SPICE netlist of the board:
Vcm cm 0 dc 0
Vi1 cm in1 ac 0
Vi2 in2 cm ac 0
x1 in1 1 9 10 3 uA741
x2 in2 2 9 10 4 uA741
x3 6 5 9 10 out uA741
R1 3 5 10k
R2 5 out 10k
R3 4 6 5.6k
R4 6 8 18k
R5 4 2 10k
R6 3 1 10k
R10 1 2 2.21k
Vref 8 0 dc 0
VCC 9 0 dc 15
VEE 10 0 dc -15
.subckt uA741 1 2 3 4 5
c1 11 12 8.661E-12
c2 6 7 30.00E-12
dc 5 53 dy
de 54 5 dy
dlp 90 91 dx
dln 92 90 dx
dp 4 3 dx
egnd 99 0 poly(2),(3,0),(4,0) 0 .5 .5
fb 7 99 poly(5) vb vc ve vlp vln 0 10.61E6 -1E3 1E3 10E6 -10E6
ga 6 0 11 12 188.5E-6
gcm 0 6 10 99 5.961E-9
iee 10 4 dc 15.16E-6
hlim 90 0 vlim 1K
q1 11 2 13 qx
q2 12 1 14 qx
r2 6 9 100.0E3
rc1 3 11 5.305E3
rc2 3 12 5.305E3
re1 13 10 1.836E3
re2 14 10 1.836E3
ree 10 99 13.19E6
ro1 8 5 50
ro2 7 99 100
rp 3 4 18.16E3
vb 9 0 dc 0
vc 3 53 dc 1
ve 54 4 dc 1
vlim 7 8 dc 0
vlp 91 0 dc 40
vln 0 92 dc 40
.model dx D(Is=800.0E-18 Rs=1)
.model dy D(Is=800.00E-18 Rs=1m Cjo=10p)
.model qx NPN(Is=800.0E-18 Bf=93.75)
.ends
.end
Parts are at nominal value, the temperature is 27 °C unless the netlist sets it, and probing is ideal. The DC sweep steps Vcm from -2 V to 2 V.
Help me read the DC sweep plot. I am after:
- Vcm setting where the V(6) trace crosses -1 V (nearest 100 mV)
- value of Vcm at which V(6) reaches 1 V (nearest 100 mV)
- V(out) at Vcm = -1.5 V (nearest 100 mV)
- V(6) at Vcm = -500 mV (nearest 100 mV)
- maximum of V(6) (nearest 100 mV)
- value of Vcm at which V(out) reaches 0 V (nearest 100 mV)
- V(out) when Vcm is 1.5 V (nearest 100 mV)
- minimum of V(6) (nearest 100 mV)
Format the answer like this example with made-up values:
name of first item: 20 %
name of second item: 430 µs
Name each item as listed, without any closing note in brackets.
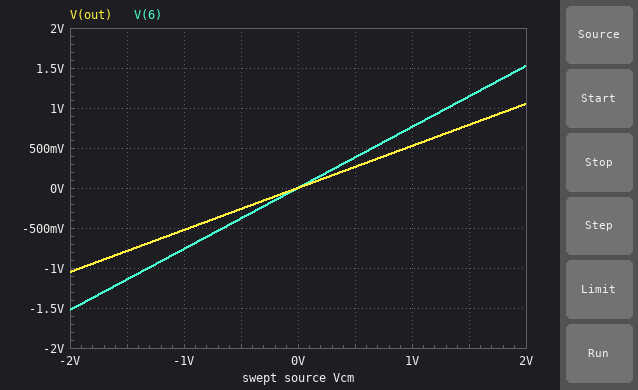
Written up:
Vcm setting where the V(6) trace crosses -1 V: -1.3 V
value of Vcm at which V(6) reaches 1 V: 1.3 V
V(out) at Vcm = -1.5 V: -800 mV
V(6) at Vcm = -500 mV: -400 mV
maximum of V(6): 1.5 V
value of Vcm at which V(out) reaches 0 V: 0 V
V(out) when Vcm is 1.5 V: 800 mV
minimum of V(6): -1.5 V
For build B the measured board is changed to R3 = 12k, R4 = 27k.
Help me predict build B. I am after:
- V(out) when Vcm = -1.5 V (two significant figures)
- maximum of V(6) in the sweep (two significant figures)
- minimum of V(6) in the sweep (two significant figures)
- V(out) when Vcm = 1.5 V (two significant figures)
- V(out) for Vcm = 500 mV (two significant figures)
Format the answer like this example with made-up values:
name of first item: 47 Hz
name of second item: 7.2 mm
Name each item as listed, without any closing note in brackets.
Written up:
V(out) when Vcm = -1.5 V: -580 mV
maximum of V(6) in the sweep: 1.4 V
minimum of V(6) in the sweep: -1.4 V
V(out) when Vcm = 1.5 V: 580 mV
V(out) for Vcm = 500 mV: 190 mV
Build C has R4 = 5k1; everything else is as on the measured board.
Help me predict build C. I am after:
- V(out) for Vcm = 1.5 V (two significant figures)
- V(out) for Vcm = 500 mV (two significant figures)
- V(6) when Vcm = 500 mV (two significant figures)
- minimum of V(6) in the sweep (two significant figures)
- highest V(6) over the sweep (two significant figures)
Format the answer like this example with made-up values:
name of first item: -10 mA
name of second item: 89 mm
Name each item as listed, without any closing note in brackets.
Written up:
V(out) for Vcm = 1.5 V: -70 mV
V(out) for Vcm = 500 mV: -23 mV
V(6) when Vcm = 500 mV: 240 mV
minimum of V(6) in the sweep: -950 mV
highest V(6) over the sweep: 950 mV
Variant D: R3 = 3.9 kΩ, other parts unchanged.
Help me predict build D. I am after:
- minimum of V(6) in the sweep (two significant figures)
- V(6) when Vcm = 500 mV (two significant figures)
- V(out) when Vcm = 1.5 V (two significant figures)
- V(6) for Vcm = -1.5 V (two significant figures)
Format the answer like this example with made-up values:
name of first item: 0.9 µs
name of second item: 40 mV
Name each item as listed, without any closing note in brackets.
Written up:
minimum of V(6) in the sweep: -1.6 V
V(6) when Vcm = 500 mV: 410 mV
V(out) when Vcm = 1.5 V: 970 mV
V(6) for Vcm = -1.5 V: -1.2 V
